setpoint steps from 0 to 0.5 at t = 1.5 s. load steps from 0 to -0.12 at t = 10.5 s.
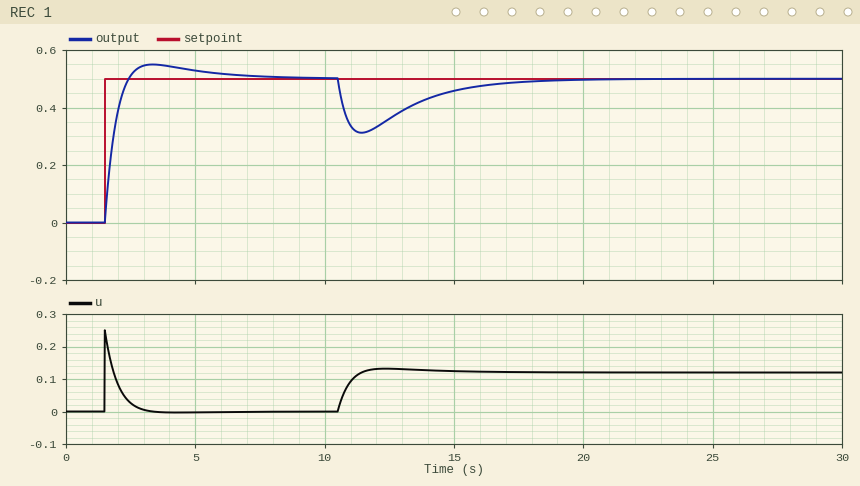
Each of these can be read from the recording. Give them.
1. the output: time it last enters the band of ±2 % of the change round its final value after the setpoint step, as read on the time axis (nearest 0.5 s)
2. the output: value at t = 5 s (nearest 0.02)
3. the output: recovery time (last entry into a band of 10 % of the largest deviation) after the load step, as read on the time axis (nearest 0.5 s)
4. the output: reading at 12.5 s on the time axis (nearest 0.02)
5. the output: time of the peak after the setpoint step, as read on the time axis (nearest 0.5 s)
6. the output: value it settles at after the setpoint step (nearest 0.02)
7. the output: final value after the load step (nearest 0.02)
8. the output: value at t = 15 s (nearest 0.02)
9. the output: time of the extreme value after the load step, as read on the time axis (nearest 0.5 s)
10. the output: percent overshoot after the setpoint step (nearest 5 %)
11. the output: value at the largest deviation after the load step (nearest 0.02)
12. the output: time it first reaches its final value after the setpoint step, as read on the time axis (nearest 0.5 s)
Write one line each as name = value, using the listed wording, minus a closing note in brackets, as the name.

the output: time it last enters the band of ±2 % of the change round its final value after the setpoint step, as read on the time axis = 7.0 s
the output: value at t = 5 s = 0.52
the output: recovery time (last entry into a band of 10 % of the largest deviation) after the load step, as read on the time axis = 16.5 s
the output: reading at 12.5 s on the time axis = 0.36
the output: time of the peak after the setpoint step, as read on the time axis = 3.5 s
the output: value it settles at after the setpoint step = 0.50
the output: final value after the load step = 0.50
the output: value at t = 15 s = 0.46
the output: time of the extreme value after the load step, as read on the time axis = 11.5 s
the output: percent overshoot after the setpoint step = 10 %
the output: value at the largest deviation after the load step = 0.32
the output: time it first reaches its final value after the setpoint step, as read on the time axis = 2.5 s
